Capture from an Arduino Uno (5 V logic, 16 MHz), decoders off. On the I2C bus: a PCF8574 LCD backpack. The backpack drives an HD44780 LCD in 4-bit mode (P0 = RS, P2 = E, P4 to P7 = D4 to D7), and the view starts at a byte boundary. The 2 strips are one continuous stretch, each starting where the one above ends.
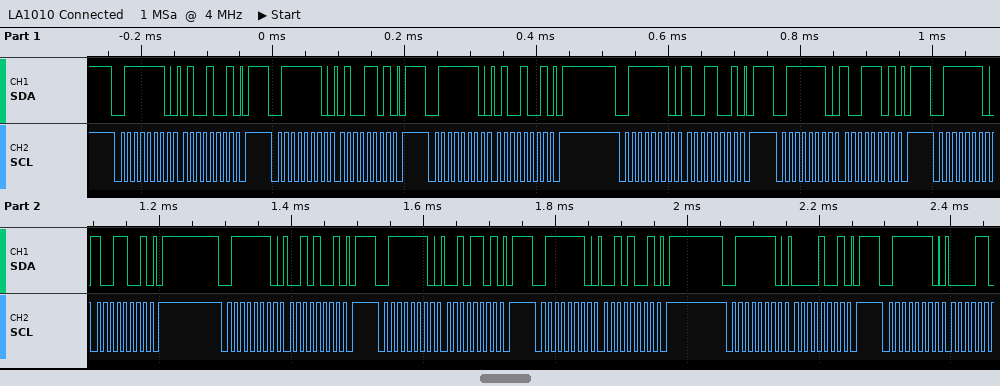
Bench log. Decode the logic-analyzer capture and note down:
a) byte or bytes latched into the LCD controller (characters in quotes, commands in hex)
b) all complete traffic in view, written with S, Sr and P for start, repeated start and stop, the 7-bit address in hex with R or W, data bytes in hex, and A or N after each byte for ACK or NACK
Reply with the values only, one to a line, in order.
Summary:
'I'
S 3FW A 49 A P S 3FW A 4D A P S 3FW A 49 A P S 3FW A 99 A P S 3FW A 9D A P S 3FW A 99 A P S 3FW A 29 A P S 3FW A 2D A P S 3FW A 29 A P S 3FW A 09 A P S 3FW A
